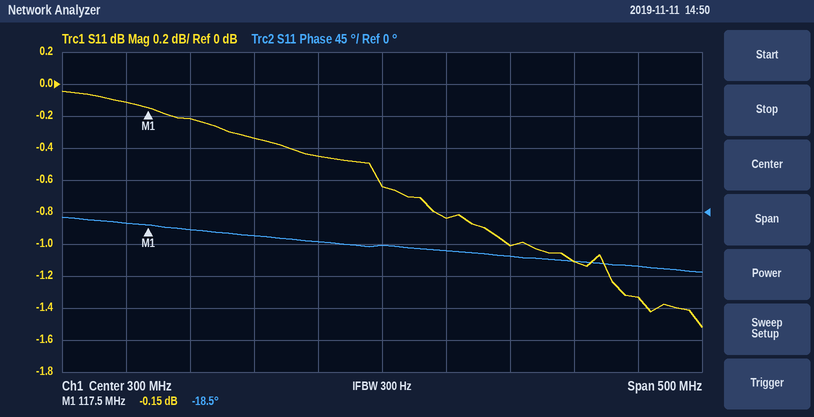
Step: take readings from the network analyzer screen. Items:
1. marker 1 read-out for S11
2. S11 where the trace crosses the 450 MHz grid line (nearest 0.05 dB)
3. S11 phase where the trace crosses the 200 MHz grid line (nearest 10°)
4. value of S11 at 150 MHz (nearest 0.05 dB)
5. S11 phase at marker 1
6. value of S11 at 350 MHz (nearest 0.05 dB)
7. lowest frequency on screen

-0.15 dB
-1.10 dB
-30°
-0.20 dB
-18.5°
-0.85 dB
50 MHz
